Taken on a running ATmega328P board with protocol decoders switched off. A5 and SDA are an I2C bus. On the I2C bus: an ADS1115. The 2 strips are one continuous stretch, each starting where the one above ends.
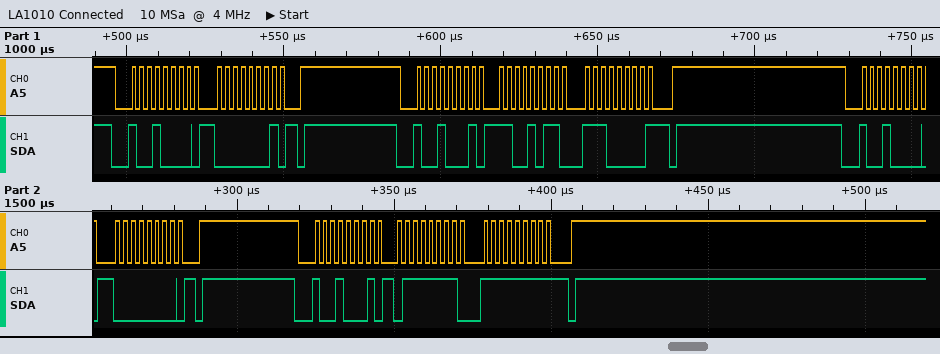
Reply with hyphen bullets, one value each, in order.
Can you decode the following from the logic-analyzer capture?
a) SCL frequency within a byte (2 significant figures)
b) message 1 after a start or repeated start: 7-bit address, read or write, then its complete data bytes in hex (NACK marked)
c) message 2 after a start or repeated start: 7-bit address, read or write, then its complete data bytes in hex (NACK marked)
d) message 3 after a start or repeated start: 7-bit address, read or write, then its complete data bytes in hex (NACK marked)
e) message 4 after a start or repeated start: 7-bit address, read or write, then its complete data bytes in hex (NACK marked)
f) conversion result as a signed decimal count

- 400 kHz
- 0x48 write: 01
- 0x48 read: CB E0 NACK
- 0x48 write: 00
- 0x48 read: 7F FF NACK
- 32767
